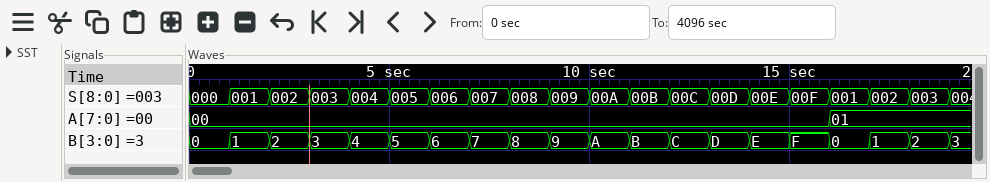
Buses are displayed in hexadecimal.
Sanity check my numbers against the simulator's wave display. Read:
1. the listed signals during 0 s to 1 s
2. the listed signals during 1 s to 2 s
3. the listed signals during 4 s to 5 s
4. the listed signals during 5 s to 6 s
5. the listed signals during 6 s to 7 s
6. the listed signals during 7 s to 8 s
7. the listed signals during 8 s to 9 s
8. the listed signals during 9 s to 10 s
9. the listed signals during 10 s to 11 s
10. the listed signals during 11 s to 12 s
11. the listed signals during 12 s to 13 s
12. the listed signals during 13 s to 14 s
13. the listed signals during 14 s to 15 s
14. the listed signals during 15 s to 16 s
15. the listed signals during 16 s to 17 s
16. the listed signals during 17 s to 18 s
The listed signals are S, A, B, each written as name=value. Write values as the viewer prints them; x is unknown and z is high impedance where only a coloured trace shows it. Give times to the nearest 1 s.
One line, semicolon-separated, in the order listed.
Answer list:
S=000, A=00, B=0; S=001, A=00, B=1; S=004, A=00, B=4; S=005, A=00, B=5; S=006, A=00, B=6; S=007, A=00, B=7; S=008, A=00, B=8; S=009, A=00, B=9; S=00A, A=00, B=A; S=00B, A=00, B=B; S=00C, A=00, B=C; S=00D, A=00, B=D; S=00E, A=00, B=E; S=00F, A=00, B=F; S=001, A=01, B=0; S=002, A=01, B=1
